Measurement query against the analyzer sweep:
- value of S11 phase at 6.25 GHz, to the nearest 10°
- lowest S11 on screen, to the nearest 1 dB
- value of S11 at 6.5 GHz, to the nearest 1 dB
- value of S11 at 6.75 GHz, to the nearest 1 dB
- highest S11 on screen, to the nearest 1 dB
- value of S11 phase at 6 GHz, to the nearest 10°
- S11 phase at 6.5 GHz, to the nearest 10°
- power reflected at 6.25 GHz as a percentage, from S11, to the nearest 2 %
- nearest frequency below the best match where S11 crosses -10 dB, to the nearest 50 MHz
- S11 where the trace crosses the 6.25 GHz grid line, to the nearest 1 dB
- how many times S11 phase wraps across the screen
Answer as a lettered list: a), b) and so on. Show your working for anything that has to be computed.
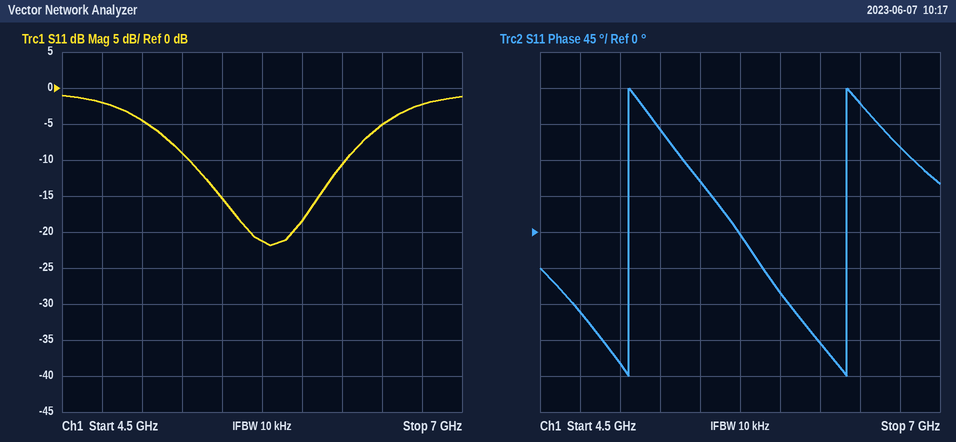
a) -140°
b) -22 dB
c) -5 dB
d) -2 dB
e) -1 dB
f) -80°
g) 160°
h) 10^(-11/10) ≈ 8 %
i) 5.30 GHz
j) -11 dB
k) 2
